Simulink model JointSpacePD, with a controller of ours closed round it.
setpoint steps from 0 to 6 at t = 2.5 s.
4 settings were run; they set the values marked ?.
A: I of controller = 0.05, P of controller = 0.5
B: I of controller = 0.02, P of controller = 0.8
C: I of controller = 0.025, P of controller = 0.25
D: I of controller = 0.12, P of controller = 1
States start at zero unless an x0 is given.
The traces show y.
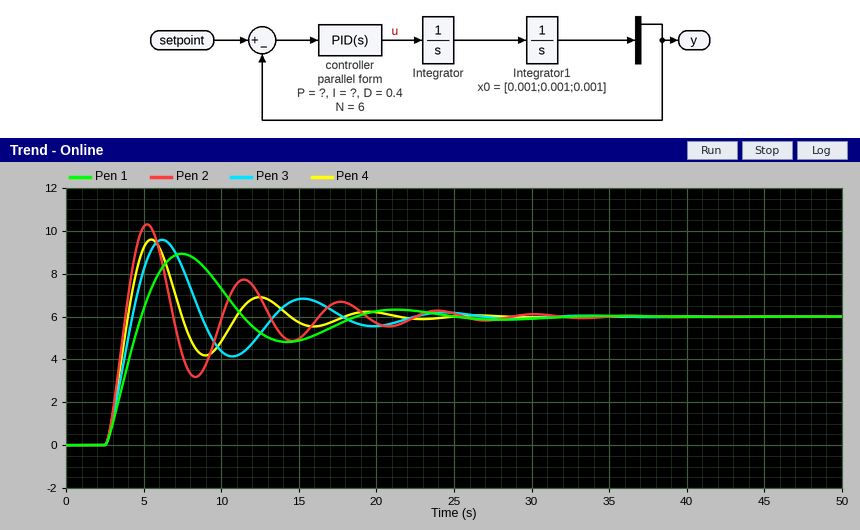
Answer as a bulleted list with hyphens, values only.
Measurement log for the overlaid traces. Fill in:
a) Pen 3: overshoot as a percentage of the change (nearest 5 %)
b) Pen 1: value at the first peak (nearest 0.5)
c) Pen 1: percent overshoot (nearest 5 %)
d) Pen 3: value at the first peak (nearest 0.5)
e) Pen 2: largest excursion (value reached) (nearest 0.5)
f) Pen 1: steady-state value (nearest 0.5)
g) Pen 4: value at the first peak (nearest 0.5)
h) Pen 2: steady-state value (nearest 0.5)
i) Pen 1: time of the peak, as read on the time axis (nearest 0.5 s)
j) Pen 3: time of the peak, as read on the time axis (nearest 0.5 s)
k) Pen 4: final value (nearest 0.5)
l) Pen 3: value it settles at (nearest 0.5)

- 60 %
- 9.0
- 50 %
- 9.5
- 10.5
- 6.0
- 9.5
- 6.0
- 7.5 s
- 6.0 s
- 6.0
- 6.0
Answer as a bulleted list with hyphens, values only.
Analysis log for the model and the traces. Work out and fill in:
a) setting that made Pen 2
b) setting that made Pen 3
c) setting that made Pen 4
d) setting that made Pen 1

- D
- A
- B
- C
